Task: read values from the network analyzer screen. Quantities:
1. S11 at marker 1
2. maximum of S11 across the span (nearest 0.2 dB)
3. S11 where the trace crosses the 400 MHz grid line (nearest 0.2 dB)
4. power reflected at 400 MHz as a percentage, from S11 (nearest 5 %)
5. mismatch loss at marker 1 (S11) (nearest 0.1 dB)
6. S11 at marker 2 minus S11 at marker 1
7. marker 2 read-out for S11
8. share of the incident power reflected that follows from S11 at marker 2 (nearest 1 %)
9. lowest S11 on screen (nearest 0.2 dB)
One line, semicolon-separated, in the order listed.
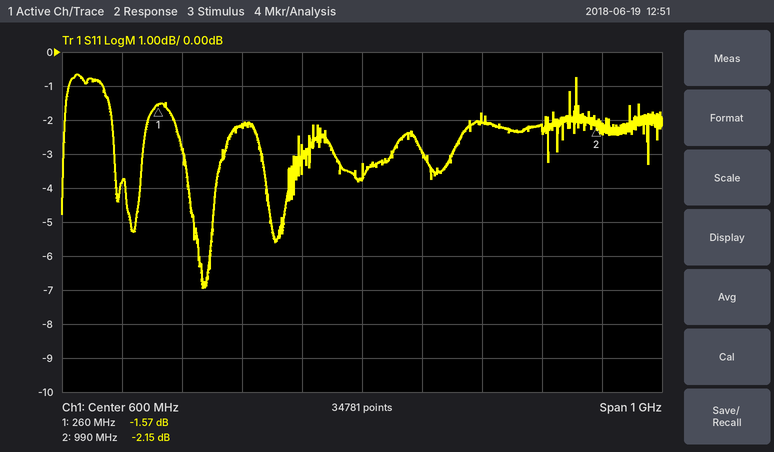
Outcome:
-1.57 dB; -0.6 dB; -2.2 dB; 60 %; 5.2 dB; -0.58 dB; -2.15 dB; 61 %; -7.0 dB
